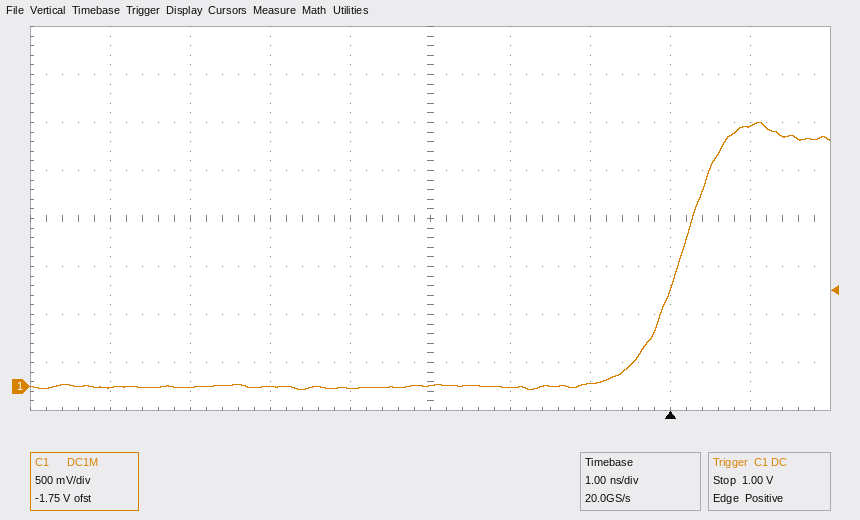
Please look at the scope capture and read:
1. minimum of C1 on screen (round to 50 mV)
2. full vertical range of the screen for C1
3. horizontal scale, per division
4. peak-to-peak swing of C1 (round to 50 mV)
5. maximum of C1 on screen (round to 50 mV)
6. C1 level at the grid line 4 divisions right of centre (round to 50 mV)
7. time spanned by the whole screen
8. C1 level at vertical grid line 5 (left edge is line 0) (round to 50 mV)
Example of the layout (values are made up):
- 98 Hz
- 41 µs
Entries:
- -50 mV
- 4 V
- 1 ns
- 2.80 V
- 2.75 V
- 2.70 V
- 10 ns
- 0 mV
